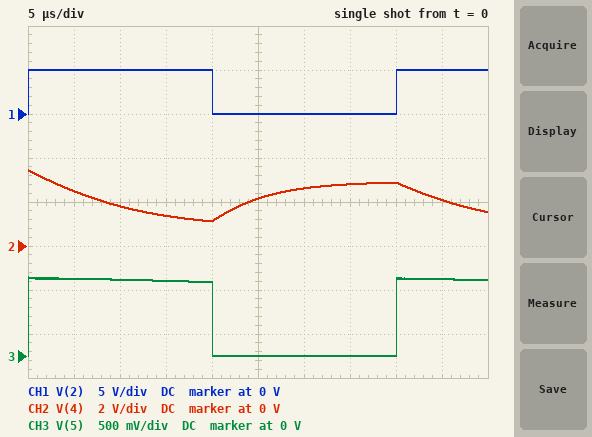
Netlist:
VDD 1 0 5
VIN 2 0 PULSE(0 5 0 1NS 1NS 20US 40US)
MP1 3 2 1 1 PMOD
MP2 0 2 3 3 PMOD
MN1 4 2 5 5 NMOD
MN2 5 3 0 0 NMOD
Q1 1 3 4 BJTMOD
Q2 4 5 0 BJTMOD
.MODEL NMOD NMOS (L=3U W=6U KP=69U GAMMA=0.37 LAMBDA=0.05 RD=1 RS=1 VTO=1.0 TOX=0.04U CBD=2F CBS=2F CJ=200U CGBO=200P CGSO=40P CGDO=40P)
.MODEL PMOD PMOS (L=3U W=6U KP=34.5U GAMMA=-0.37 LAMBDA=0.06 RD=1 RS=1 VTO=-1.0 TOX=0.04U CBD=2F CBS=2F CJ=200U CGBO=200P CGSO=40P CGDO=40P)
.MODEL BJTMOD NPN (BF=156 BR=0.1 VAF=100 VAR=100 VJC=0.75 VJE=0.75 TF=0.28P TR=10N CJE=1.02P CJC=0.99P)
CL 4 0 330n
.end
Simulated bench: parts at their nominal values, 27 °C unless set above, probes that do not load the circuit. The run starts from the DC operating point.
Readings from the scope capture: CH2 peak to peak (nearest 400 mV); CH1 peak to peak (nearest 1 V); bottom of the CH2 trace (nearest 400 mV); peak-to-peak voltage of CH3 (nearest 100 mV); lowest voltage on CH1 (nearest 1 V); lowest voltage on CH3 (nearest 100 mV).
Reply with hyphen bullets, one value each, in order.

- 2.4 V
- 5 V
- 1.2 V
- 900 mV
- 0 V
- 0 V
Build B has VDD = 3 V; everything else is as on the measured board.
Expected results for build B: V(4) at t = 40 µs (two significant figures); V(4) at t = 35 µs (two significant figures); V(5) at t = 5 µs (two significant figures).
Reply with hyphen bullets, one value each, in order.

- 1.5 V
- 1.4 V
- 860 mV
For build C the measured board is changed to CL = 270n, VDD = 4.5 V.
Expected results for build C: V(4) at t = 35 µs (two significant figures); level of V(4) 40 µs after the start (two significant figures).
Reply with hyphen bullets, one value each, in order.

- 2.5 V
- 2.6 V
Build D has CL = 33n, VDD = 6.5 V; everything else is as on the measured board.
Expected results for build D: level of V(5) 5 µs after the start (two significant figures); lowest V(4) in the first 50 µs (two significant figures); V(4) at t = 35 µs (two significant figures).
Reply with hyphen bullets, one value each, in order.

- 800 mV
- 890 mV
- 4.0 V
